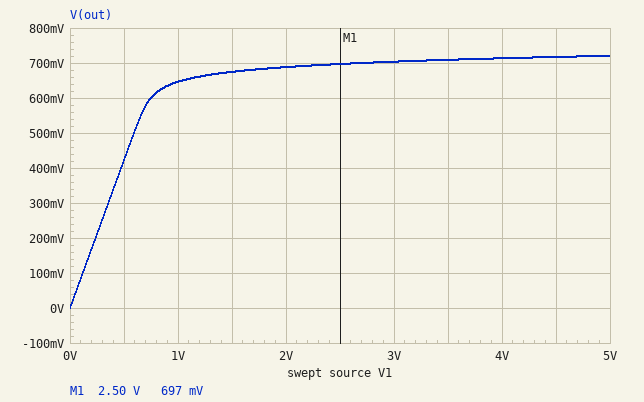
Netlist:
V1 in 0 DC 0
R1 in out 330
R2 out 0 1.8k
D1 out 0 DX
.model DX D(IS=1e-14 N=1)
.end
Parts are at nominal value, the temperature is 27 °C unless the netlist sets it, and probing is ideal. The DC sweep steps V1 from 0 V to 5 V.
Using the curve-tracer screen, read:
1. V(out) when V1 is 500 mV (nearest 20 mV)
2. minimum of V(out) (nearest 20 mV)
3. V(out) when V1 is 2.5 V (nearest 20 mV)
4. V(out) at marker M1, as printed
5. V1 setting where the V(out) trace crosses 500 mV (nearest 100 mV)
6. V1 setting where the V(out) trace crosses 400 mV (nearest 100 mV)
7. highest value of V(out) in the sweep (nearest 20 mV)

420 mV
0 V
700 mV
697 mV
600 mV
500 mV
720 mV
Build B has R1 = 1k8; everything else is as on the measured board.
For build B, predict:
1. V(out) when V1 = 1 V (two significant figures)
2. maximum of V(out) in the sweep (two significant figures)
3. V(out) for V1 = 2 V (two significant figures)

500 mV
670 mV
630 mV
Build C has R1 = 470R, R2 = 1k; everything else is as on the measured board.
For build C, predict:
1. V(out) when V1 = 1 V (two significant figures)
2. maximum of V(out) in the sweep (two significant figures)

610 mV
710 mV
